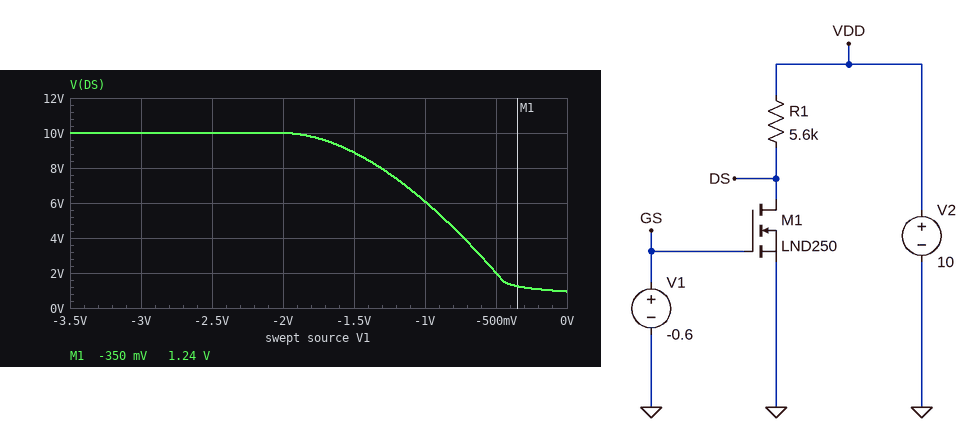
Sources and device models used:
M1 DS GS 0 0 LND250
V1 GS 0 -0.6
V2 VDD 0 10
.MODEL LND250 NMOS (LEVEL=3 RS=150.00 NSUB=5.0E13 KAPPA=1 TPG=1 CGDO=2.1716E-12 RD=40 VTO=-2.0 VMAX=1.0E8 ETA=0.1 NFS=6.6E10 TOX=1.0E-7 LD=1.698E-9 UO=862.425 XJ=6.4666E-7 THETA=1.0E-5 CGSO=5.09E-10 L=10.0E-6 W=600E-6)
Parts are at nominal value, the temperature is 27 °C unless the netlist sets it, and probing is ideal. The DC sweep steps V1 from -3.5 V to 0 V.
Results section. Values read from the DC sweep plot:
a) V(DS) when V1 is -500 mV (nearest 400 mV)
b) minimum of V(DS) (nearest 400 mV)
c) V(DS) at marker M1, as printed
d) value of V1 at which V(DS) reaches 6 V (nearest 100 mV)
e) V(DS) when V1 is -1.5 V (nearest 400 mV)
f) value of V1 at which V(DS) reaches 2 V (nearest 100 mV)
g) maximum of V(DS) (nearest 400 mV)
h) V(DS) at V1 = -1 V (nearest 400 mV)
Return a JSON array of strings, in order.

["2.0 V", "800 mV", "1.24 V", "-1.0 V", "8.8 V", "-500 mV", "10.0 V", "6.0 V"]
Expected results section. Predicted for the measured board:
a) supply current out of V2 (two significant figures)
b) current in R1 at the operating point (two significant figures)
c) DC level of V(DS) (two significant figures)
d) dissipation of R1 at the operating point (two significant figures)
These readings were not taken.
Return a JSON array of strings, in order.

["1.3 mA", "1.3 mA", "2.9 V", "9.0 mW"]
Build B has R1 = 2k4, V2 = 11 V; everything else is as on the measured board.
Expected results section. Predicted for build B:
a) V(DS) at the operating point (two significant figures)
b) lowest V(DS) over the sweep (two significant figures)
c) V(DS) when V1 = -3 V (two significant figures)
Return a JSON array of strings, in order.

["8.0 V", "5.4 V", "11 V"]
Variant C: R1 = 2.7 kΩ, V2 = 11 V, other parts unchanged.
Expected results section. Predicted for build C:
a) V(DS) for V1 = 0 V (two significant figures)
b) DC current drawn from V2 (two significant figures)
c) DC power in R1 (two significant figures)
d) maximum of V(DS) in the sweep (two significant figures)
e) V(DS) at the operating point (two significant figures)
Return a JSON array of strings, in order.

["4.7 V", "1.3 mA", "4.3 mW", "11 V", "7.6 V"]
